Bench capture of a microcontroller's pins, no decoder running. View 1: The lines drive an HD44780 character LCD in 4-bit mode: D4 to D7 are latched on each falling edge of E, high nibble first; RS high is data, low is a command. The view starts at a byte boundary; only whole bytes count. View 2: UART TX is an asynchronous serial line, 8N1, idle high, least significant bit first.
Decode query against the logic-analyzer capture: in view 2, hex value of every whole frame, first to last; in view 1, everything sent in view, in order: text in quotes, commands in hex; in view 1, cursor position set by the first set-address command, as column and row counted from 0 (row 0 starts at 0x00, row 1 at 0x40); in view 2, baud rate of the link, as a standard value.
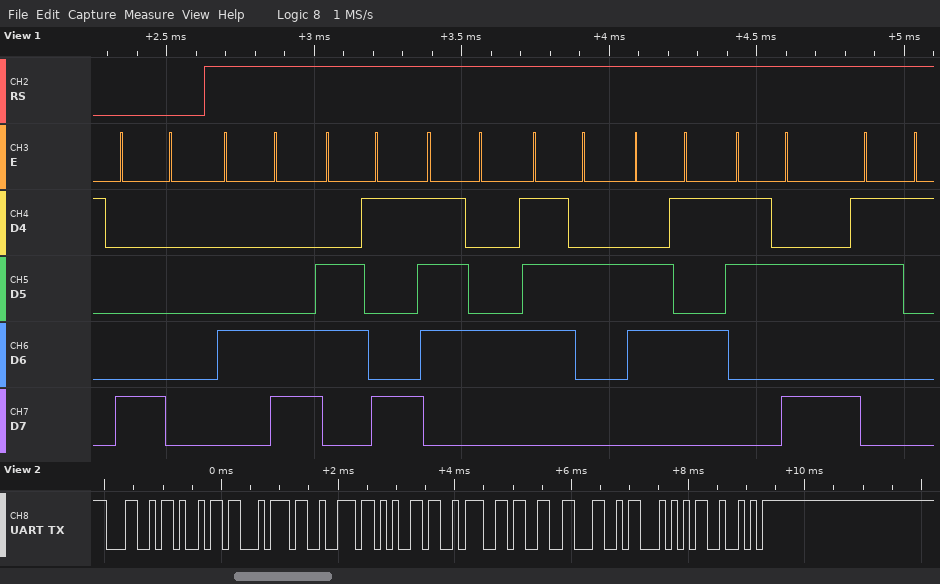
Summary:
0x4C 0x69 0x74 0x72 0x65 0x3A 0x33 0x4C 0x54 0x52
0x80 "Litre:1"
column 0, row 0
9600 baud
